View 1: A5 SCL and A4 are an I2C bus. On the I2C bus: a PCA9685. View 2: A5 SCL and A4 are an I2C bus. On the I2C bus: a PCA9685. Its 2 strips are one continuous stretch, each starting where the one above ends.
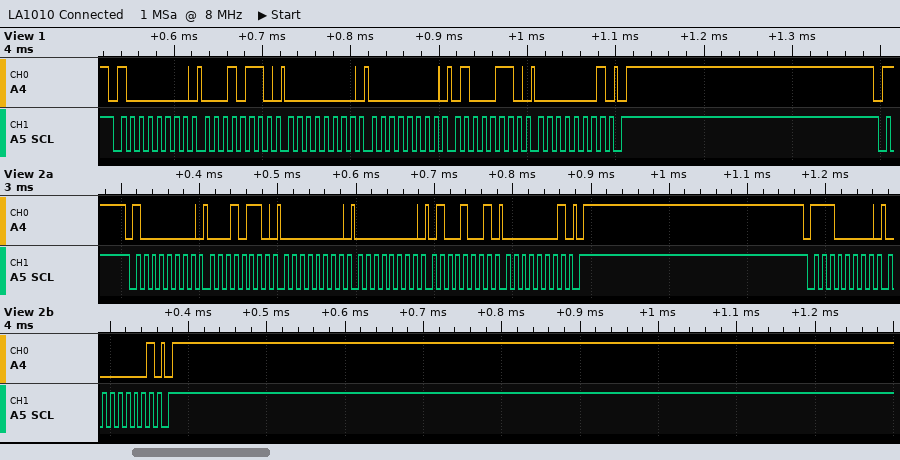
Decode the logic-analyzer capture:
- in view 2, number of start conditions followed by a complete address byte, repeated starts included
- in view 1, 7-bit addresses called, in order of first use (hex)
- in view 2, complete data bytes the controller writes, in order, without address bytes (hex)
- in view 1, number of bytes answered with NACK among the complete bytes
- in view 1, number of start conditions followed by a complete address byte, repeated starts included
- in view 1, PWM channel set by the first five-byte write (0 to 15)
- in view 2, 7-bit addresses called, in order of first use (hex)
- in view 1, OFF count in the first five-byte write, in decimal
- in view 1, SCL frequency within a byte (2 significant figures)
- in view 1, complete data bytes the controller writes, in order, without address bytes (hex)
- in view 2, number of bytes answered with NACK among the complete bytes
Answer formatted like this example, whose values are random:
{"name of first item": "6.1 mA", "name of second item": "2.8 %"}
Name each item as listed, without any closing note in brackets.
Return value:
{"in view 2, number of start conditions followed by a complete address byte, repeated starts included": "2", "in view 1, 7-bit addresses called, in order of first use": "0x40", "in view 2, complete data bytes the controller writes, in order, without address bytes": "16 00 00 49 01 01", "in view 1, number of bytes answered with NACK among the complete bytes": "0", "in view 1, number of start conditions followed by a complete address byte, repeated starts included": "1", "in view 1, PWM channel set by the first five-byte write": "4", "in view 2, 7-bit addresses called, in order of first use": "0x40 0x70", "in view 1, OFF count in the first five-byte write, in decimal": "326", "in view 1, SCL frequency within a byte": "100 kHz", "in view 1, complete data bytes the controller writes, in order, without address bytes": "16 00 00 46 01", "in view 2, number of bytes answered with NACK among the complete bytes": "0"}
